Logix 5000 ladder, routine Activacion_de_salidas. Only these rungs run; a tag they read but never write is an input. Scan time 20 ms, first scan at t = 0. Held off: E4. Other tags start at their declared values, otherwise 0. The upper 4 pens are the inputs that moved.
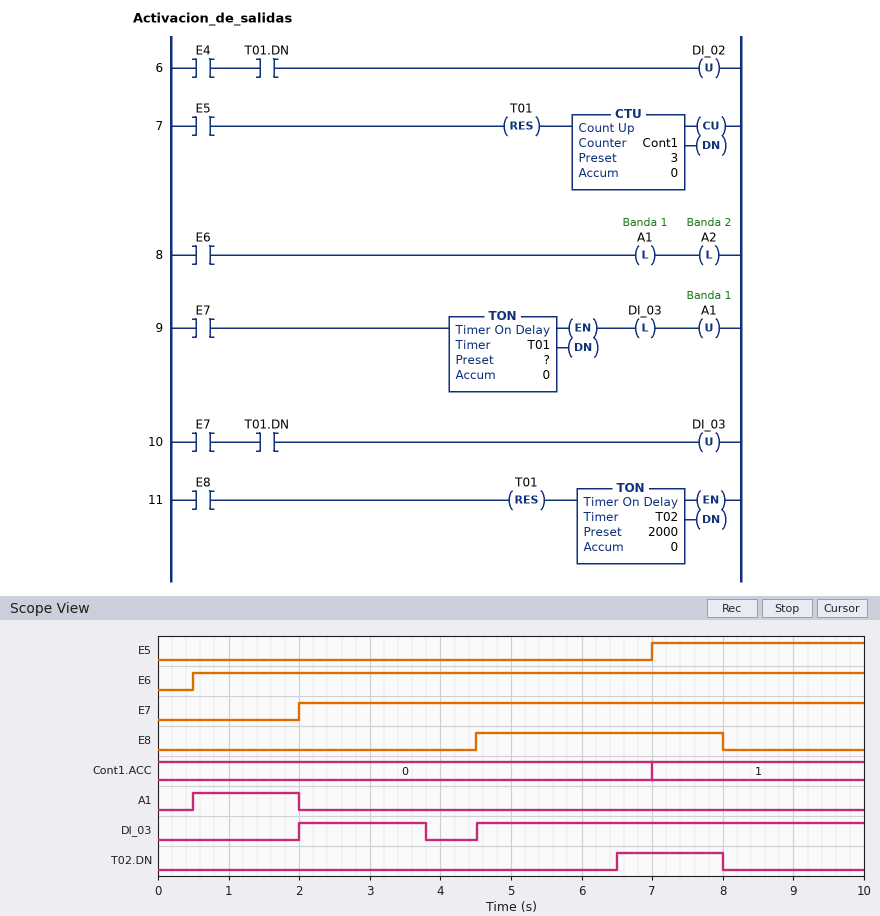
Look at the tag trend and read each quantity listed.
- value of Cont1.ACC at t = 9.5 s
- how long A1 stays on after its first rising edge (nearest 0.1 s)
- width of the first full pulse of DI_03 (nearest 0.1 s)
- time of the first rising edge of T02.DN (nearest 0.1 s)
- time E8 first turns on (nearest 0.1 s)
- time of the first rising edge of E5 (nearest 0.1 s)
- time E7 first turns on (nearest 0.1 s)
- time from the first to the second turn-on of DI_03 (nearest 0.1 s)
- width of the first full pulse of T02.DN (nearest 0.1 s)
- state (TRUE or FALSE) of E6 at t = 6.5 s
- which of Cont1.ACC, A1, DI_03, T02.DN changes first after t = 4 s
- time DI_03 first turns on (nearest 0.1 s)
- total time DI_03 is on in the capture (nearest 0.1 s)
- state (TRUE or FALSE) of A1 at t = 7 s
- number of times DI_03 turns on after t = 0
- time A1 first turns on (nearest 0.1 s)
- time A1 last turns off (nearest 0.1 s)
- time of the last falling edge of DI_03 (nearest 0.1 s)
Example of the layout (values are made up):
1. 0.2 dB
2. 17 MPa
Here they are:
1. 1
2. 1.5 s
3. 1.8 s
4. 6.5 s
5. 4.5 s
6. 7.0 s
7. 2.0 s
8. 2.5 s
9. 1.5 s
10. TRUE
11. DI_03
12. 2.0 s
13. 7.3 s
14. FALSE
15. 2
16. 0.5 s
17. 2.0 s
18. 3.8 s
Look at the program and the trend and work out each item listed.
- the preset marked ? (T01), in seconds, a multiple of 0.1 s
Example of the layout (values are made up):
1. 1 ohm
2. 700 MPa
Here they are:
1. 1.8 s
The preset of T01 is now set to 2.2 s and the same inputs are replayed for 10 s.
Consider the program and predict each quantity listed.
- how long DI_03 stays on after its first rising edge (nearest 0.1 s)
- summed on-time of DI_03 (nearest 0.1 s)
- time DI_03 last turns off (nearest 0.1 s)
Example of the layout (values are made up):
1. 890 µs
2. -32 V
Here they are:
1. 2.2 s
2. 7.7 s
3. 4.2 s
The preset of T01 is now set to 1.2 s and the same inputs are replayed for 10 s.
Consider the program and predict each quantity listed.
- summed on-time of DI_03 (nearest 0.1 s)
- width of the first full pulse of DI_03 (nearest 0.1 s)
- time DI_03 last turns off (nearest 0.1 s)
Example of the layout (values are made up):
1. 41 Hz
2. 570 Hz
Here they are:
1. 6.7 s
2. 1.2 s
3. 3.2 s
